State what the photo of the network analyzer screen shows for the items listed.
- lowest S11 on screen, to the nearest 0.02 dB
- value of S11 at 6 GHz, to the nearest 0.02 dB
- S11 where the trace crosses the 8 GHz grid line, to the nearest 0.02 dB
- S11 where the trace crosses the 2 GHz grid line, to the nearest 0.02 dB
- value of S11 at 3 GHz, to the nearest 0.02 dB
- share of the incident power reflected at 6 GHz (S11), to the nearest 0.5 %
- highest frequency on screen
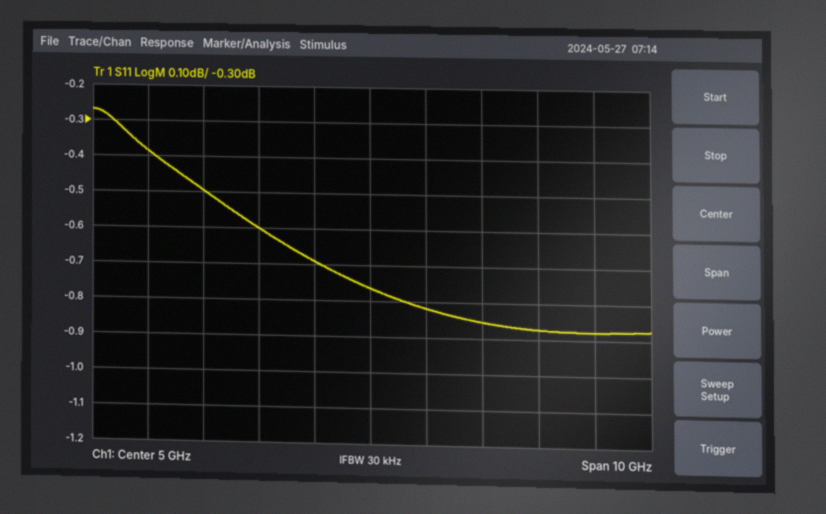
-0.88 dB
-0.82 dB
-0.88 dB
-0.50 dB
-0.60 dB
83.0 %
10 GHz
